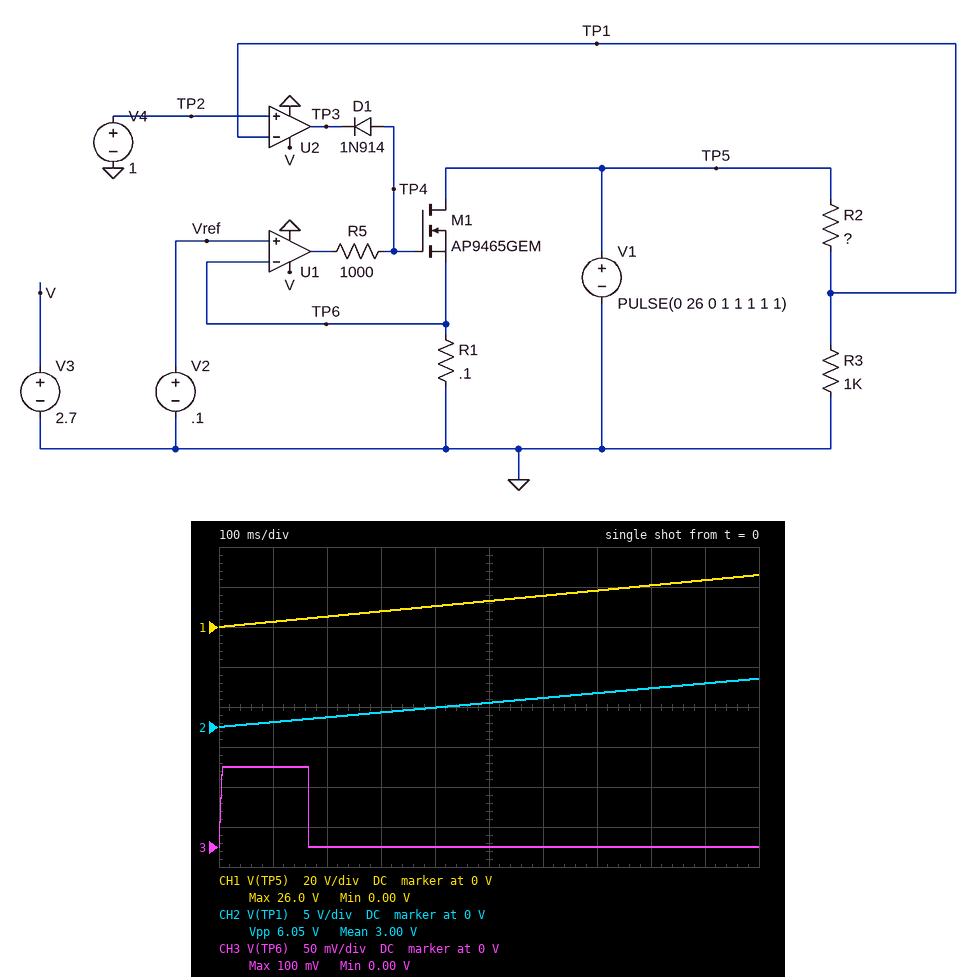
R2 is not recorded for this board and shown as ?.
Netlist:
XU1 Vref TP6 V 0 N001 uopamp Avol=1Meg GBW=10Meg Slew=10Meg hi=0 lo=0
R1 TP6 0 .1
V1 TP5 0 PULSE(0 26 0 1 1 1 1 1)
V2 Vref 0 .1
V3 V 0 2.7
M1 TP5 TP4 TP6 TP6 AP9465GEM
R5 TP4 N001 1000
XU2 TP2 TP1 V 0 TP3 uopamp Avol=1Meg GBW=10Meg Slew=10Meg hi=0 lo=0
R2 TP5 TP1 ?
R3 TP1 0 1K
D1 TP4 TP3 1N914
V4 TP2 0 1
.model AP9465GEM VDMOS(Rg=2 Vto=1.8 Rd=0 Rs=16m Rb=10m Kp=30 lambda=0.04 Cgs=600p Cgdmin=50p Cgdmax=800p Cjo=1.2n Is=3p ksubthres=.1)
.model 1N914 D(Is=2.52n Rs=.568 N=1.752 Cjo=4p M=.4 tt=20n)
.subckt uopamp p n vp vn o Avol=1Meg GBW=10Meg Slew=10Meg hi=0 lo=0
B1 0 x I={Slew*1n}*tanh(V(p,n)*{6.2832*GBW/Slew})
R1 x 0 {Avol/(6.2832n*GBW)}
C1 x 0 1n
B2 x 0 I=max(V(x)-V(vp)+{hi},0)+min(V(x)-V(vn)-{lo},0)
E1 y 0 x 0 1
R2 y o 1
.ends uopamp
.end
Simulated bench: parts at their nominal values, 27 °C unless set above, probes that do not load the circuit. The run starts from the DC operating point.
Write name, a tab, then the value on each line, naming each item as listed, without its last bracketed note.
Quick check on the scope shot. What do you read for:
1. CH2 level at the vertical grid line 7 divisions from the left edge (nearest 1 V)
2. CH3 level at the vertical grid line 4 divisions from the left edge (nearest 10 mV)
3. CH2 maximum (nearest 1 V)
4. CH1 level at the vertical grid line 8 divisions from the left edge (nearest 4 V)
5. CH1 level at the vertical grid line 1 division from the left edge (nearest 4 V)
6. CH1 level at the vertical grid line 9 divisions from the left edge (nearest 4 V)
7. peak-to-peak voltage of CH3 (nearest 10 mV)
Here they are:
CH2 level at the vertical grid line 7 divisions from the left edge	4 V
CH3 level at the vertical grid line 4 divisions from the left edge	0 V
CH2 maximum	6 V
CH1 level at the vertical grid line 8 divisions from the left edge	20 V
CH1 level at the vertical grid line 1 division from the left edge	4 V
CH1 level at the vertical grid line 9 divisions from the left edge	24 V
peak-to-peak voltage of CH3	100 mV
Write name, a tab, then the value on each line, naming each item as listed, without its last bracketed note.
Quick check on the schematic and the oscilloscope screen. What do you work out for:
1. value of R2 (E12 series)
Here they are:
value of R2	3.3 kΩ
